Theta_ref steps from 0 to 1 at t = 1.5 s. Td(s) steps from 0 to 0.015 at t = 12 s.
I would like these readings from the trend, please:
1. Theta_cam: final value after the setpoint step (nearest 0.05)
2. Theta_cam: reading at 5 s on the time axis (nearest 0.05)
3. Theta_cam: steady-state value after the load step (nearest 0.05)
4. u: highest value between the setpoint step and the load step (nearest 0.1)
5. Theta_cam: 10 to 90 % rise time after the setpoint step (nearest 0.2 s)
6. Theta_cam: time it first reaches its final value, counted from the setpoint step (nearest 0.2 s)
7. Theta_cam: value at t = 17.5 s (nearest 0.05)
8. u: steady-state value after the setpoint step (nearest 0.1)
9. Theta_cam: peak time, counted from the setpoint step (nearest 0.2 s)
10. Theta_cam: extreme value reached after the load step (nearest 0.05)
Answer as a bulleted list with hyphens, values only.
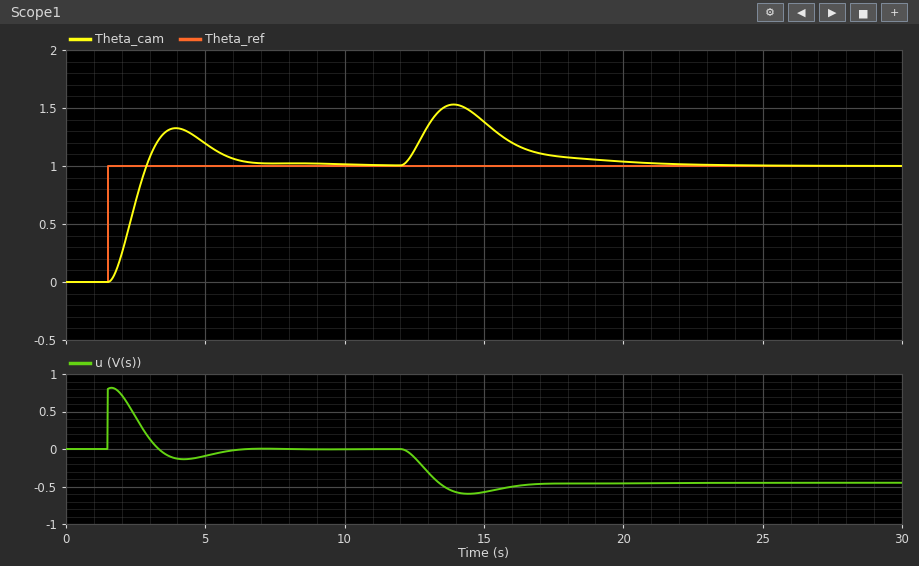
- 1.00
- 1.20
- 1.00
- 0.8
- 1.0 s
- 1.4 s
- 1.10
- 0.0
- 2.4 s
- 1.55
